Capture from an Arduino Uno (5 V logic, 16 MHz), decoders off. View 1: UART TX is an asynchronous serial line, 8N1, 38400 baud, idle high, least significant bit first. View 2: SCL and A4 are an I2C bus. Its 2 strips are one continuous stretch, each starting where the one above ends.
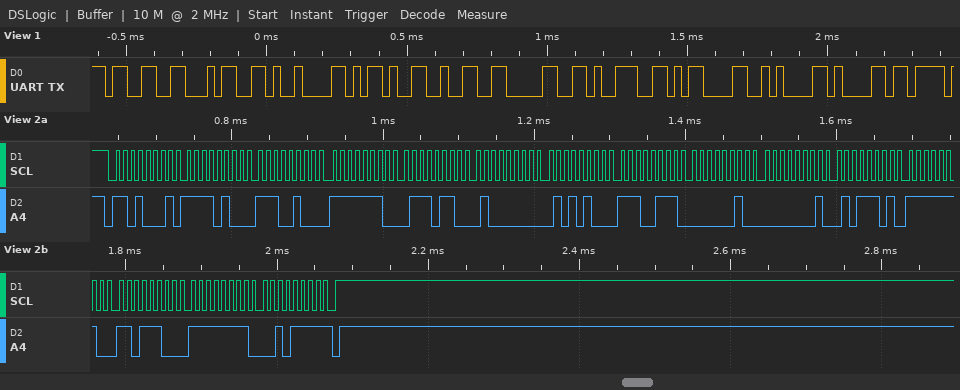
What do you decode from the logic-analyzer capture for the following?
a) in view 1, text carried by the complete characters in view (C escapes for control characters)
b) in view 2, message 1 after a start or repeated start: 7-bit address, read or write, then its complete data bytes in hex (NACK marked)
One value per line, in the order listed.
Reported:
"34\t-209\r\na"
0x68 read: F4 E4 FE 76 40 54 E7 02 01 5D FE DC FF 2F NACK
